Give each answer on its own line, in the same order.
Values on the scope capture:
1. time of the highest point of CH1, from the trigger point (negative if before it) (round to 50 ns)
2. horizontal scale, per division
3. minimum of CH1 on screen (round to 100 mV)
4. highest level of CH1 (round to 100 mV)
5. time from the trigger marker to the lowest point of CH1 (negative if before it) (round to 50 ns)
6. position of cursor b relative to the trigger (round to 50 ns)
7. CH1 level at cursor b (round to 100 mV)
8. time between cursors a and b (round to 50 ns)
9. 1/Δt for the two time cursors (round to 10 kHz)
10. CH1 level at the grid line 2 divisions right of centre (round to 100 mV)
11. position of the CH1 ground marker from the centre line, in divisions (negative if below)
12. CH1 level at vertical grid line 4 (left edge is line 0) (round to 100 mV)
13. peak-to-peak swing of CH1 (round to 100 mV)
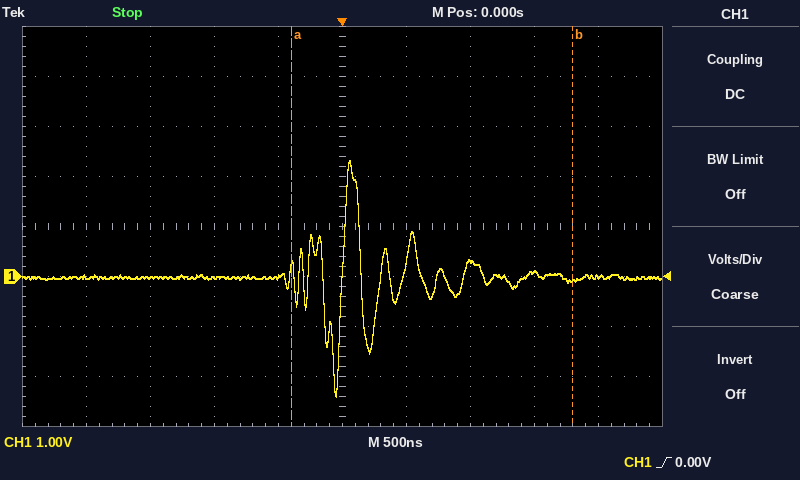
+50 ns
500 ns
-2.4 V
2.3 V
-50 ns
+1.80 µs
-100 mV
2.20 µs
450 kHz
300 mV
-1.0 div
0.0 V
4.7 V
